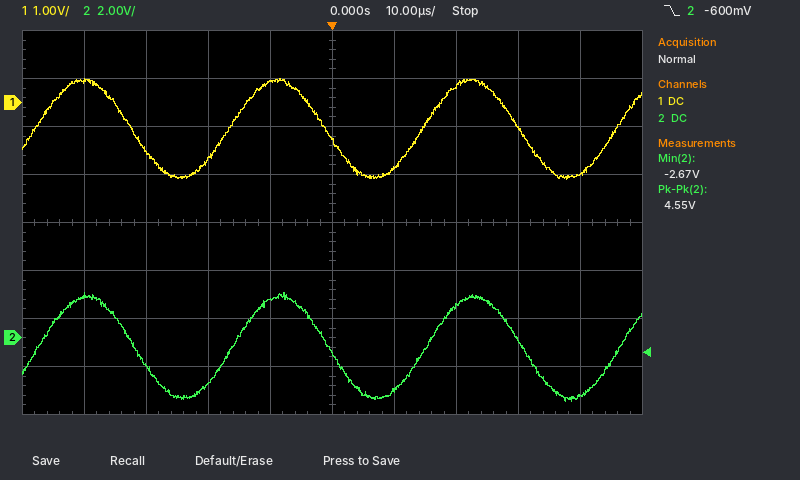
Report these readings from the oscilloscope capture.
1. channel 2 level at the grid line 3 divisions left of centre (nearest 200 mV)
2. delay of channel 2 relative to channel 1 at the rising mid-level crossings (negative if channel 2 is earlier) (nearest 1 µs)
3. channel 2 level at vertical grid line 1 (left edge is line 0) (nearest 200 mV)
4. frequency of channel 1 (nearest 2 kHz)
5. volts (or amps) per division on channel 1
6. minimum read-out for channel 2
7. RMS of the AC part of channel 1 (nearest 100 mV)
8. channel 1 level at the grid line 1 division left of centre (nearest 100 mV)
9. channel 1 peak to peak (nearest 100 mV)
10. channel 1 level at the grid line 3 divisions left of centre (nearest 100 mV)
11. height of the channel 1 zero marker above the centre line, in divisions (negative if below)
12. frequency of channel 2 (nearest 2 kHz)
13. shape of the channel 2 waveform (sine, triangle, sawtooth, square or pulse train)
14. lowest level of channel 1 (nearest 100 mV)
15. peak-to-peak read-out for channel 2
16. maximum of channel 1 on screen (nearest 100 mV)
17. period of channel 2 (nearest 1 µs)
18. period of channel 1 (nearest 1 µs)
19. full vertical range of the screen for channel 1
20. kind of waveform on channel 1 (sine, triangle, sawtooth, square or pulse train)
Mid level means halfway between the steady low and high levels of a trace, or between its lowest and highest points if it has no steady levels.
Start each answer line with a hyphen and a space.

- -1.2 V
- +1 µs
- 1.8 V
- 32 kHz
- 1 V
- -2.67 V
- 700 mV
- 400 mV
- 2.1 V
- -1.0 V
- +2.5 div
- 32 kHz
- sine
- -1.6 V
- 4.55 V
- 500 mV
- 31 µs
- 31 µs
- 8 V
- sine
